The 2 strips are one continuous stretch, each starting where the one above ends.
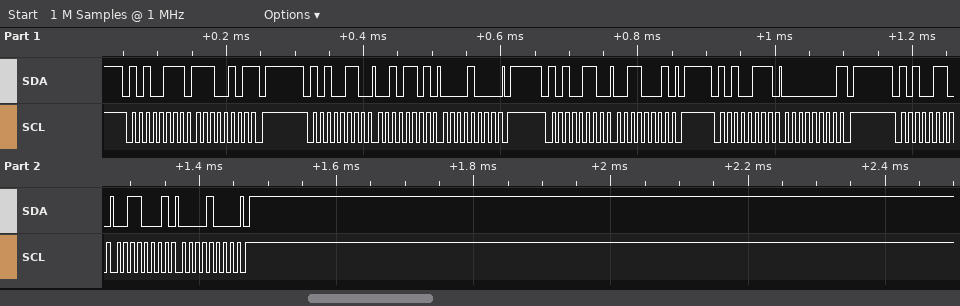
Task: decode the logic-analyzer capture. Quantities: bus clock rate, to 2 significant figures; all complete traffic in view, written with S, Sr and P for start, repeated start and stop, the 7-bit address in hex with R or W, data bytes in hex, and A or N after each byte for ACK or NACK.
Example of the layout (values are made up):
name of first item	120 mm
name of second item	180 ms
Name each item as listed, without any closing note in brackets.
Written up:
bus clock rate, to 2 significant figures	100 kHz
all complete traffic in view, written with S, Sr and P for start, repeated start and stop, the 7-bit address in hex with R or W, data bytes in hex, and A or N after each byte for ACK or NACK	S 53R A E5 N P S 53W A 2D A 08 A P S 53W A 31 A P S 53R A 00 N P S 53W A 31 A 08 A P
